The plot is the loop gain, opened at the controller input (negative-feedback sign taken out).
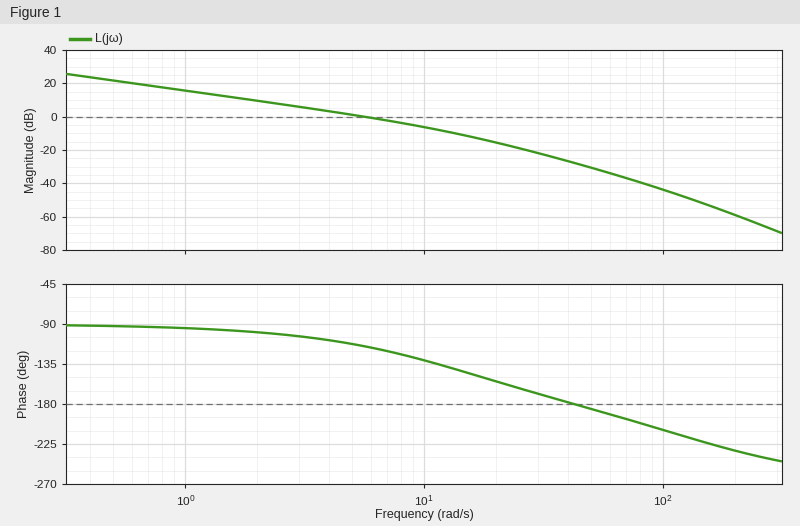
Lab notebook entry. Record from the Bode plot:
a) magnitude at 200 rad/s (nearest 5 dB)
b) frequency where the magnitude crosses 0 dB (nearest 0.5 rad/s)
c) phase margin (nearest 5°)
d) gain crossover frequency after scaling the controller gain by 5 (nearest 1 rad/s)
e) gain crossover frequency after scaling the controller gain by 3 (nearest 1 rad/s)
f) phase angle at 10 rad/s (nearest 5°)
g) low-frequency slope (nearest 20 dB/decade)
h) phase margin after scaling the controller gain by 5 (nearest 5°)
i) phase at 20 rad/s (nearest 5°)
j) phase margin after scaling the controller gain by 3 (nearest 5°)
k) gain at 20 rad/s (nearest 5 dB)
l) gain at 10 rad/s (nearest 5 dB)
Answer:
-60 dB
5.5 rad/s
65°
18 rad/s
13 rad/s
-130°
-20 dB/decade
30°
-155°
40°
-15 dB
-5 dB
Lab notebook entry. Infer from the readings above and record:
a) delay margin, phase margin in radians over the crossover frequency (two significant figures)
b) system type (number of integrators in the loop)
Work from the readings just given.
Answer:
0.21 s
1
